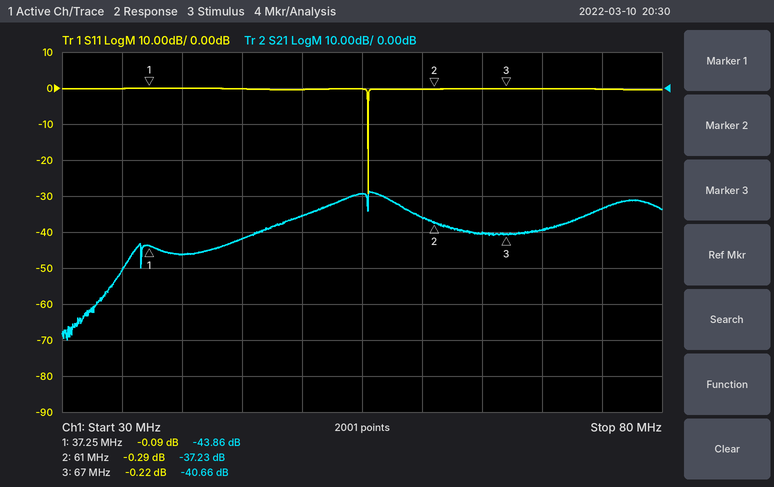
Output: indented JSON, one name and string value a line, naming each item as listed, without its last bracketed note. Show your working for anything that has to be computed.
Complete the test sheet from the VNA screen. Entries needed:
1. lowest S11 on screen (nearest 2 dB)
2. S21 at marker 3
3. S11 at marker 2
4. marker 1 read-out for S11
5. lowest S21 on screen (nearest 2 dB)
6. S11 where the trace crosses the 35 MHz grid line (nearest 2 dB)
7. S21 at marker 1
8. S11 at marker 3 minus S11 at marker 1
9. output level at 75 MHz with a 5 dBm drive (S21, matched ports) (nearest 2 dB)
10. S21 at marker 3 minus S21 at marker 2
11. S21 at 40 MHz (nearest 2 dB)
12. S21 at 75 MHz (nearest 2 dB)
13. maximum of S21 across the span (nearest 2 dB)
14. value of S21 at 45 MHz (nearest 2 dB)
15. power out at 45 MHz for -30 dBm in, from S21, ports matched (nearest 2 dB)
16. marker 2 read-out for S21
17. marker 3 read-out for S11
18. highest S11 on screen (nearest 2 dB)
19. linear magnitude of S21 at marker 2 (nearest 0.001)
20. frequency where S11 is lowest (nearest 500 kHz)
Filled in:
{
  "lowest S11 on screen": "-30 dB",
  "S21 at marker 3": "-40.66 dB",
  "S11 at marker 2": "-0.29 dB",
  "marker 1 read-out for S11": "-0.09 dB",
  "lowest S21 on screen": "-70 dB",
  "S11 where the trace crosses the 35 MHz grid line": "0 dB",
  "S21 at marker 1": "-43.86 dB",
  "S11 at marker 3 minus S11 at marker 1": "-0.22 − (-0.09) = -0.13 dB",
  "output level at 75 MHz with a 5 dBm drive (S21, matched ports)": "5 dBm + (-34 dB) = -28 dBm",
  "S21 at marker 3 minus S21 at marker 2": "-40.66 − (-37.23) = -3.43 dB",
  "S21 at 40 MHz": "-46 dB",
  "S21 at 75 MHz": "-34 dB",
  "maximum of S21 across the span": "-28 dB",
  "value of S21 at 45 MHz": "-42 dB",
  "power out at 45 MHz for -30 dBm in, from S21, ports matched": "-30 dBm + (-42 dB) = -72 dBm",
  "marker 2 read-out for S21": "-37.23 dB",
  "marker 3 read-out for S11": "-0.22 dB",
  "highest S11 on screen": "0 dB",
  "linear magnitude of S21 at marker 2": "10^(-37.23/20) ≈ 0.014",
  "frequency where S11 is lowest": "55.5 MHz"
}
